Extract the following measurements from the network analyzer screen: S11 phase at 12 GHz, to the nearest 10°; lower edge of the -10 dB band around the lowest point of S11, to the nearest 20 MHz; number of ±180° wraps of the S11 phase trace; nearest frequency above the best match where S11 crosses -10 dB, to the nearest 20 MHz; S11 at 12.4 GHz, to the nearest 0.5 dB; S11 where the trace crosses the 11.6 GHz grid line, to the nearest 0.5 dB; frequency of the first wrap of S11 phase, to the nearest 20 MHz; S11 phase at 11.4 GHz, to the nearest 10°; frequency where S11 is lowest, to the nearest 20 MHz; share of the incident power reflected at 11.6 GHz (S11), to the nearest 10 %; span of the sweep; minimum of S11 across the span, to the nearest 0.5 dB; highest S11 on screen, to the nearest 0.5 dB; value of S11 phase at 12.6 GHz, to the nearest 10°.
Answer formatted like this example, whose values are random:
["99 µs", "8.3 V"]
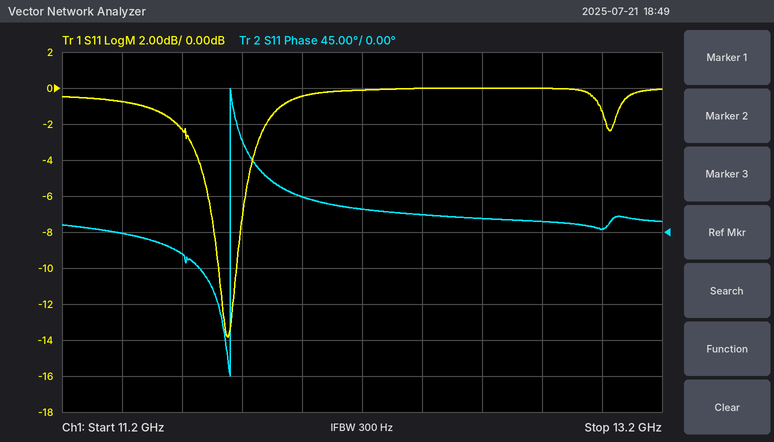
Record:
["40°", "11.72 GHz", "1", "11.78 GHz", "0.0 dB", "-2.5 dB", "11.76 GHz", "0°", "11.76 GHz", "60 %", "2 GHz", "-14.0 dB", "0.0 dB", "20°"]
